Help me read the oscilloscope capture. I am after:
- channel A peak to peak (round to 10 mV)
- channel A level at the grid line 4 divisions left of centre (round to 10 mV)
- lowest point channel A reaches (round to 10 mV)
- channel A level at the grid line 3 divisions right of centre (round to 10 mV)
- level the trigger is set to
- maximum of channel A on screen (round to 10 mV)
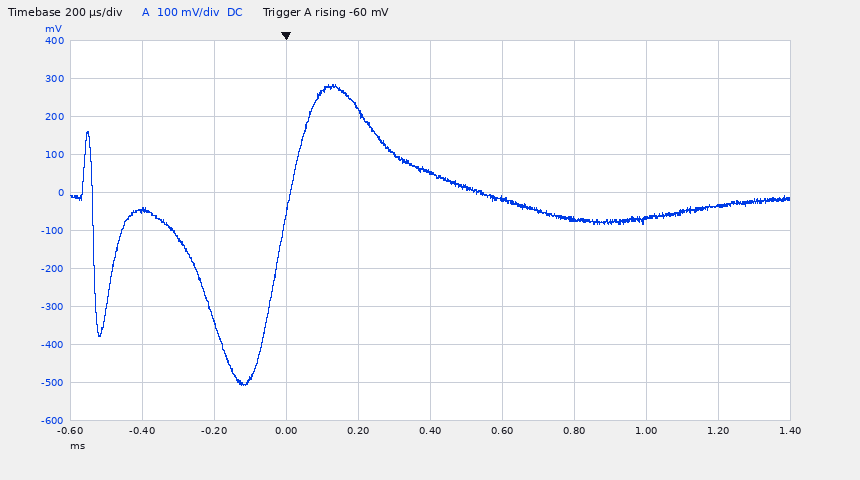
790 mV
-50 mV
-510 mV
-70 mV
-60 mV
280 mV
